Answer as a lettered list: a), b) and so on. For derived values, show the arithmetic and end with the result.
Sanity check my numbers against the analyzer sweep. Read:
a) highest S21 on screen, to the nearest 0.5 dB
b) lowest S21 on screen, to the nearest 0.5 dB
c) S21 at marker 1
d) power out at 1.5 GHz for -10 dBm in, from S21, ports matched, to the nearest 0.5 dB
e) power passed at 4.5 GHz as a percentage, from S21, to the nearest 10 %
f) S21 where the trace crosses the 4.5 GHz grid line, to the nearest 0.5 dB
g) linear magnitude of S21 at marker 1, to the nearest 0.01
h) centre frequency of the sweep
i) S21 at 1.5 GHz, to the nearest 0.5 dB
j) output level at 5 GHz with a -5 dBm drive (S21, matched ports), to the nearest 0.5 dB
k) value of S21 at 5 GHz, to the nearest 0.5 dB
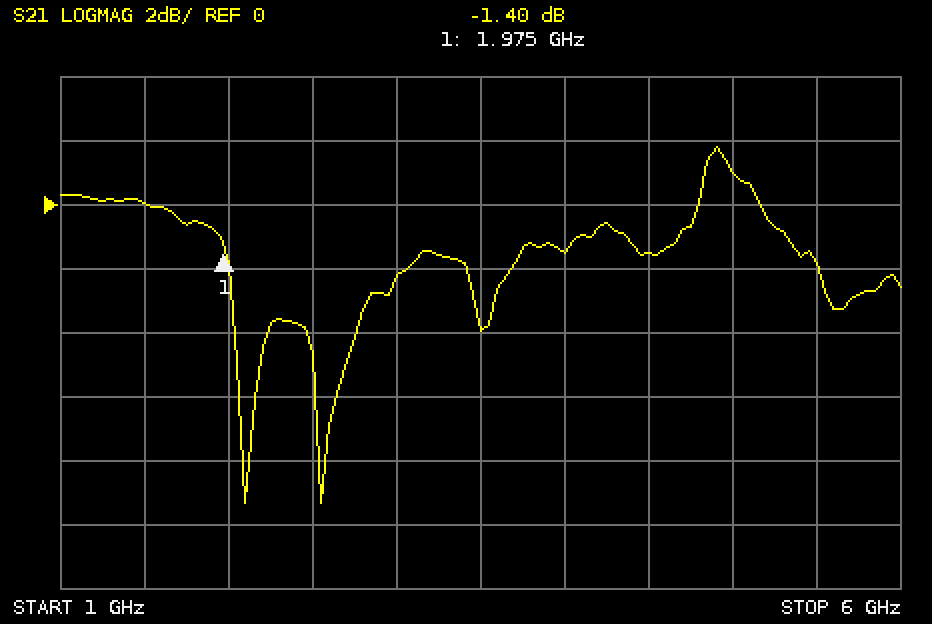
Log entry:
a) 2.0 dB
b) -9.5 dB
c) -1.40 dB
d) -10 dBm + (0.0 dB) = -10.0 dBm
e) 10^(-1.5/10) ≈ 70.8 %, so 70 % to the nearest 10 %
f) -1.5 dB
g) 10^(-1.4/20) ≈ 0.85
h) 3.5 GHz
i) 0.0 dB
j) -5 dBm + (1.0 dB) = -4.0 dBm
k) 1.0 dB
